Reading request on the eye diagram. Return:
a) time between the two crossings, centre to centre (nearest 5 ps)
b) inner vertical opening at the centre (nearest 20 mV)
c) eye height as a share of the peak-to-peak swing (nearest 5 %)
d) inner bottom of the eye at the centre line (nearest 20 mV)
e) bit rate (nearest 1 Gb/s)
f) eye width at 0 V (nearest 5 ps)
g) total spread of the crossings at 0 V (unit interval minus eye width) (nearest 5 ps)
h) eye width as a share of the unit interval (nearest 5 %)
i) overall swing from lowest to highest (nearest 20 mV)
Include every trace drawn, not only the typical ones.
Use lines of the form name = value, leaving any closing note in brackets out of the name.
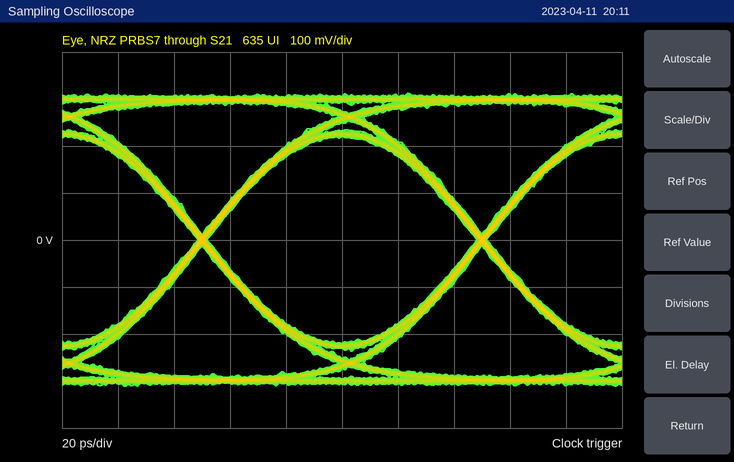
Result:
time between the two crossings, centre to centre = 100 ps
inner vertical opening at the centre = 440 mV
eye height as a share of the peak-to-peak swing = 70 %
inner bottom of the eye at the centre line = -220 mV
bit rate = 10 Gb/s
eye width at 0 V = 95 ps
total spread of the crossings at 0 V (unit interval minus eye width) = 5 ps
eye width as a share of the unit interval = 95 %
overall swing from lowest to highest = 620 mV
